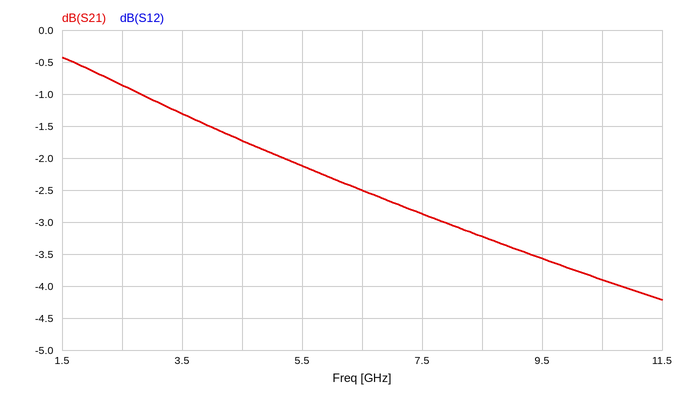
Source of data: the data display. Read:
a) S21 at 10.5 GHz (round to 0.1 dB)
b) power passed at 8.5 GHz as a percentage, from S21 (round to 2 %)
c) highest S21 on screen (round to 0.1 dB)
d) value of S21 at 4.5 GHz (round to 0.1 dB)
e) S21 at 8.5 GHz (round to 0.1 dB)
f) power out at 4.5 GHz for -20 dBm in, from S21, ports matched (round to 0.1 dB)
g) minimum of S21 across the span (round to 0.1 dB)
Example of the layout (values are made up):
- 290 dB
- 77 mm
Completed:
- -3.9 dB
- 48 %
- -0.4 dB
- -1.7 dB
- -3.2 dB
- -21.7 dBm
- -4.2 dB
